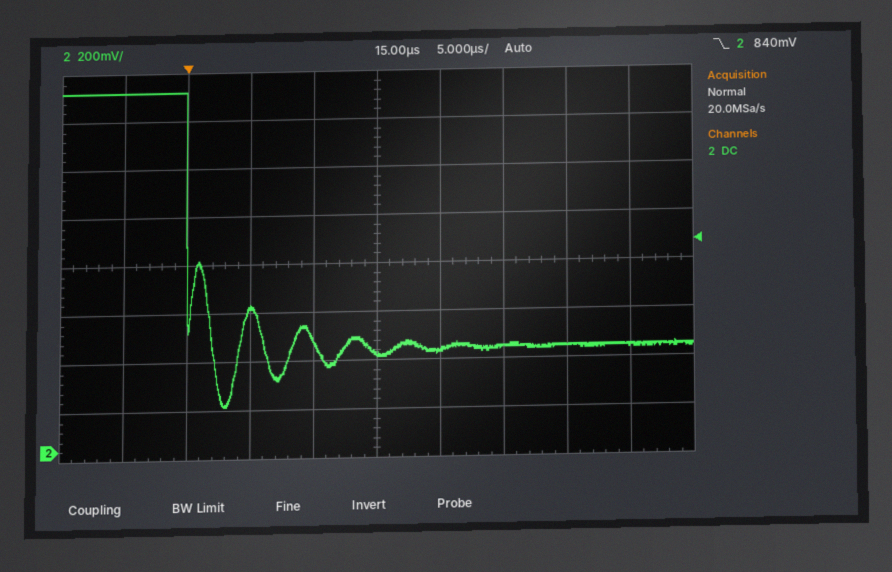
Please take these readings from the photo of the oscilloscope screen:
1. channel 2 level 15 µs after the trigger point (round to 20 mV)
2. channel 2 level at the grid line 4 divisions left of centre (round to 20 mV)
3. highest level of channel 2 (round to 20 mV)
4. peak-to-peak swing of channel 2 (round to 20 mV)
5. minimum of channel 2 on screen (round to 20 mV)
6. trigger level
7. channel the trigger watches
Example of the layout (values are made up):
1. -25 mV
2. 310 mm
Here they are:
1. 380 mV
2. 1.48 V
3. 1.48 V
4. 1.30 V
5. 180 mV
6. 840 mV
7. channel 2
